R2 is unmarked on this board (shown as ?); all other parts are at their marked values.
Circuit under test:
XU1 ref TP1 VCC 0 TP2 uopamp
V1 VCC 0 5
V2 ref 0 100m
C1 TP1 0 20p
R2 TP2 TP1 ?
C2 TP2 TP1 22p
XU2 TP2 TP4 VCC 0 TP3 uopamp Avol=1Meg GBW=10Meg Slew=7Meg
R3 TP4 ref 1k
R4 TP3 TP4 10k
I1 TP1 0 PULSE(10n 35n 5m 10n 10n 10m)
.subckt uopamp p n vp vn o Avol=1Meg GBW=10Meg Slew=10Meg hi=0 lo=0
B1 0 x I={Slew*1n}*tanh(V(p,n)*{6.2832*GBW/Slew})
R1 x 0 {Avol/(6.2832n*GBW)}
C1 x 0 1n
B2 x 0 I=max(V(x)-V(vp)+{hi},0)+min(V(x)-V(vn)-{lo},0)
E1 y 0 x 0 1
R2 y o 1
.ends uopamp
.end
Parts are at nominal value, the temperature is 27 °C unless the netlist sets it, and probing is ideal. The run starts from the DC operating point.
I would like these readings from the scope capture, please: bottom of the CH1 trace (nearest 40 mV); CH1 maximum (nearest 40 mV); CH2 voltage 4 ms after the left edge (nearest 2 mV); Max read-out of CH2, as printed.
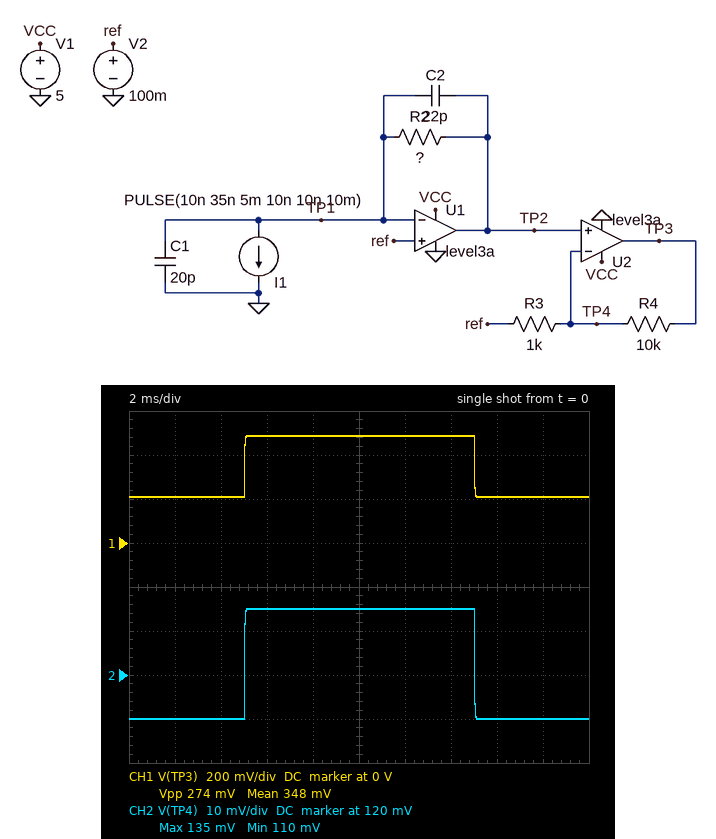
200 mV
480 mV
110 mV
135 mV
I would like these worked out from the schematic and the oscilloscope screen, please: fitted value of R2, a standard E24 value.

1 MΩ
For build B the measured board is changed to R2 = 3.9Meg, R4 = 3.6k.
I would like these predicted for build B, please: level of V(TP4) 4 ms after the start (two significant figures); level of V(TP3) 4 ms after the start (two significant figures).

140 mV
280 mV
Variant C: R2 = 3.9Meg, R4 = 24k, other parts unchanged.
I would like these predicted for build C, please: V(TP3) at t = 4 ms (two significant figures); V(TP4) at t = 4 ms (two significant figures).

1.1 V
140 mV
